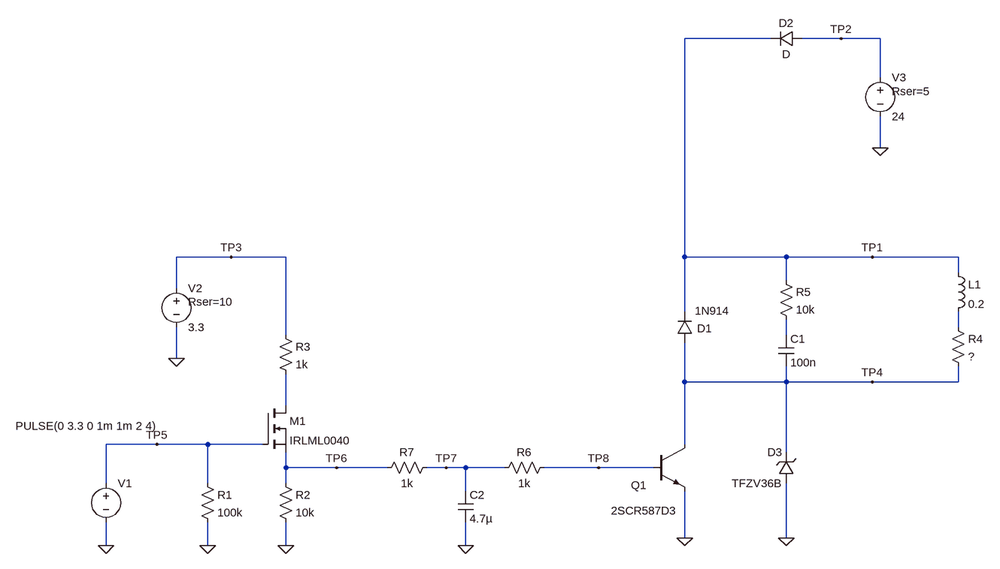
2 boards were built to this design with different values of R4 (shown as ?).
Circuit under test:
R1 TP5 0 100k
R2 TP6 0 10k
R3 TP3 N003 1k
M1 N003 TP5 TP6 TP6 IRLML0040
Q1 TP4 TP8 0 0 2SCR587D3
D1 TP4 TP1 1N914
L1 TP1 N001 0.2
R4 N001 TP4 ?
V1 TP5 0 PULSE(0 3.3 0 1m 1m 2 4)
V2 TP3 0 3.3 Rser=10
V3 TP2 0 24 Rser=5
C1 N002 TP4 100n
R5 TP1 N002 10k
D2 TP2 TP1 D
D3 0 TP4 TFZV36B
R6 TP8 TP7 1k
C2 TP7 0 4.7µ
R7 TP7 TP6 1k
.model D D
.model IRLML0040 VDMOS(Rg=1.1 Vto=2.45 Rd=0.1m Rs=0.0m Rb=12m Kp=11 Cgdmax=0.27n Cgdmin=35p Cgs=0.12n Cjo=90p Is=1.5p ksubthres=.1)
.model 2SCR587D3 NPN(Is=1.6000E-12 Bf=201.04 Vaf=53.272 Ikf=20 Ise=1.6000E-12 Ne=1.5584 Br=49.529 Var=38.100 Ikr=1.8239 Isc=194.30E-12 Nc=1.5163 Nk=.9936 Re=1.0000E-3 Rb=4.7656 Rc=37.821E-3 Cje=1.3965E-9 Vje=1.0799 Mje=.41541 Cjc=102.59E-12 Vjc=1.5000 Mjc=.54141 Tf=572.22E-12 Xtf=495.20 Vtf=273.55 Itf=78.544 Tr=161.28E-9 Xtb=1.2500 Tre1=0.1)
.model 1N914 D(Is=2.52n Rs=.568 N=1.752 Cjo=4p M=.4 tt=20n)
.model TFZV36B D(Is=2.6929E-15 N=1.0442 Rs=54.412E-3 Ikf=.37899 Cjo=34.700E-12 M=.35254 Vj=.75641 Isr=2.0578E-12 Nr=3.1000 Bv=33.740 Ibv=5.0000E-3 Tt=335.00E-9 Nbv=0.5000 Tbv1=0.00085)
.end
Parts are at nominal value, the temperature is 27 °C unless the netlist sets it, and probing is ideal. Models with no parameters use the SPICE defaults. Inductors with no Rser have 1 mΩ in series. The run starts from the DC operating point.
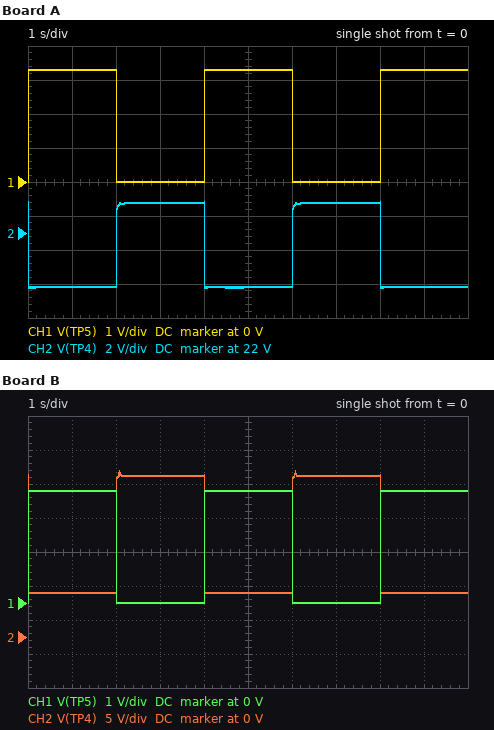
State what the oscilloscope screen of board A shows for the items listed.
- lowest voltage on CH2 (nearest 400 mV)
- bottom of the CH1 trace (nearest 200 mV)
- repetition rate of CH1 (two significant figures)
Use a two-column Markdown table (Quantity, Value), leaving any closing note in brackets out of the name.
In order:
| Quantity | Value |
|---|---|
| lowest voltage on CH2 | 18.8 V |
| bottom of the CH1 trace | 0 V |
| repetition rate of CH1 | 250 mHz |
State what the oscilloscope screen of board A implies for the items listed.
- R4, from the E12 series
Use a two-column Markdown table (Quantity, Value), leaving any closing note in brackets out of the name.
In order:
| Quantity | Value |
|---|---|
| R4, from the E12 series | 68 Ω |
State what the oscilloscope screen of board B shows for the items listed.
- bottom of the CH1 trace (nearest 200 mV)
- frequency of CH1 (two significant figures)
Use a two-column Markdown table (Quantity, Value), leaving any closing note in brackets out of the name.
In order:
| Quantity | Value |
|---|---|
| bottom of the CH1 trace | 0 V |
| frequency of CH1 | 250 mHz |
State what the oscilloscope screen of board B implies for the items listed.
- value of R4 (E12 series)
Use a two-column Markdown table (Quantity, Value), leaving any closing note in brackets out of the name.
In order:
| Quantity | Value |
|---|---|
| value of R4 | 330 Ω |
